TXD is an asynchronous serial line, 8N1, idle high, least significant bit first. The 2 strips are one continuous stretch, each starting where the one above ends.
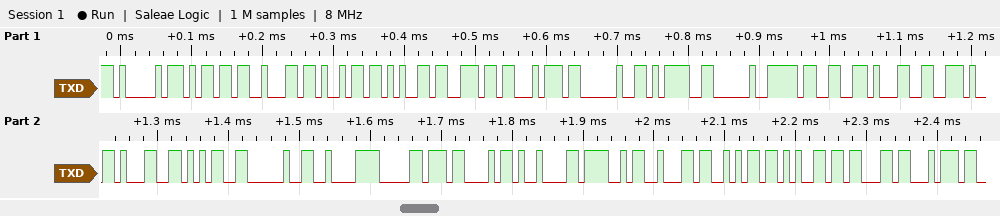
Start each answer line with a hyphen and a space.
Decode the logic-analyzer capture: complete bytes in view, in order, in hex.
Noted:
- 41 6D 62 69 65 6E 74 20 3D 20 33 31 2E 31 35 20 C2 B0 43 09 4F 62 6A 65 63 74
